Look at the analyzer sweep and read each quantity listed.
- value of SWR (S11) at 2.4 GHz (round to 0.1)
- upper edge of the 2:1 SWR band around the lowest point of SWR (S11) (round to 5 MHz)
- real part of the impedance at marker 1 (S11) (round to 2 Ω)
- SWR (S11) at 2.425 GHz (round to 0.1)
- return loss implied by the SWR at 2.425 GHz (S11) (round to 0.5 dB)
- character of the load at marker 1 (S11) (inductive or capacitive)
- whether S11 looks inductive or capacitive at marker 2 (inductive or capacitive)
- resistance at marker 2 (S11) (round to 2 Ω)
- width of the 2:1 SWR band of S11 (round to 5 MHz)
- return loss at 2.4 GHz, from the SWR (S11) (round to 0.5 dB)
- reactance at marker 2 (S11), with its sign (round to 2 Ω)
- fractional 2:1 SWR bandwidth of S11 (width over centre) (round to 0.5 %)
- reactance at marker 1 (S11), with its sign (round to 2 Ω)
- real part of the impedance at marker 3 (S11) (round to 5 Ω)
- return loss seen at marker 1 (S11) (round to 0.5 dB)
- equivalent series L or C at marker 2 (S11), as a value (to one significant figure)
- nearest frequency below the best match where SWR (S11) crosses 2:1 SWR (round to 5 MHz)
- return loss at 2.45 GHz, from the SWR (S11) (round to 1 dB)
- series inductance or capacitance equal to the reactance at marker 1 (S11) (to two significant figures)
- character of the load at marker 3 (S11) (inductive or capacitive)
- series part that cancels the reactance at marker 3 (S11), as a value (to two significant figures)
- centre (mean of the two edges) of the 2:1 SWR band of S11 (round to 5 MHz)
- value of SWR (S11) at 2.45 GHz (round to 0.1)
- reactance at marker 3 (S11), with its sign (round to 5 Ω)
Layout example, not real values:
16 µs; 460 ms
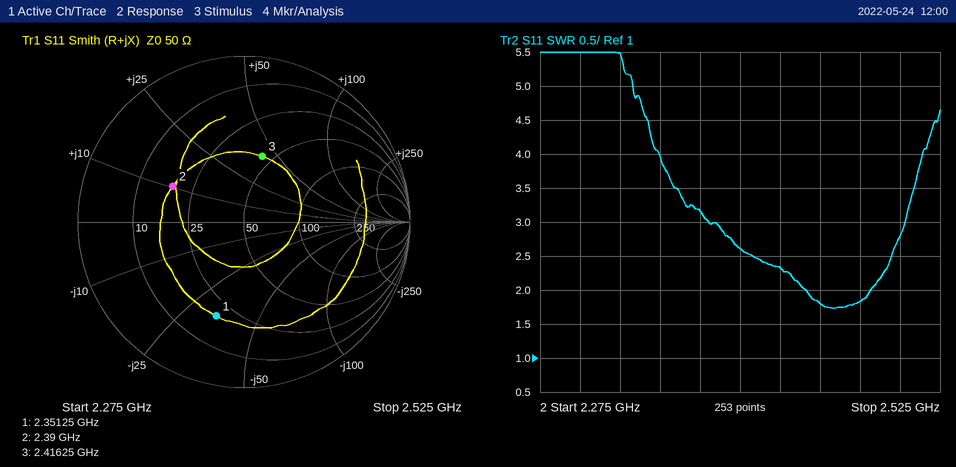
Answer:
2.6; 2.480 GHz; 20 Ω; 2.3; 8.0 dB; capacitive; inductive; 18 Ω; 40 MHz; 7.0 dB; +10 Ω; 1.5 %; -34 Ω; 45 Ω; 4.5 dB; 700 pH; 2.440 GHz; 11 dB; 2.0 pF; inductive; 1.6 pF; 2.460 GHz; 1.8; +40 Ω
